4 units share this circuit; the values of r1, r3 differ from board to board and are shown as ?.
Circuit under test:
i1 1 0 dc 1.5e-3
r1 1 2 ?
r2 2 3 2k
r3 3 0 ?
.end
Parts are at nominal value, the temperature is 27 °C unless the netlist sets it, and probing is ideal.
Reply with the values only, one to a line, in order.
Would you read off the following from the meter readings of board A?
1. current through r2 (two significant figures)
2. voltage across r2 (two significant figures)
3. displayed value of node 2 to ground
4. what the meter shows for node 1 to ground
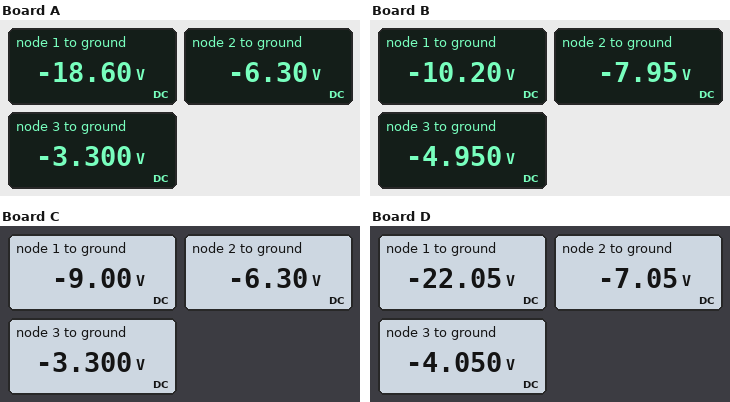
1.5 mA
3.0 V
-6.30 V
-18.60 V
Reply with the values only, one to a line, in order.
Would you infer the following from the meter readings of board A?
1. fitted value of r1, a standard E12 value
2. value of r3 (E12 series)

8.2 kΩ
2.2 kΩ
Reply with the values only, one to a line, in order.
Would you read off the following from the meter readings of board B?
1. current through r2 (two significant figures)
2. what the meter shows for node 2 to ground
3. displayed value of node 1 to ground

1.5 mA
-7.95 V
-10.20 V
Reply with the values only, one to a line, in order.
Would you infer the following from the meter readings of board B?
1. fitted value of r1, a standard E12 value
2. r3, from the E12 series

1.5 kΩ
3.3 kΩ
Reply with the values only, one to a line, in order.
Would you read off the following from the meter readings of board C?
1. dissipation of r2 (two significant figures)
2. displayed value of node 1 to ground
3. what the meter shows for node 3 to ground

4.5 mW
-9.00 V
-3.300 V
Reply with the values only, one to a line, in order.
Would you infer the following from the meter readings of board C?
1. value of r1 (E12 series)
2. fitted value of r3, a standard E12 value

1.8 kΩ
2.2 kΩ
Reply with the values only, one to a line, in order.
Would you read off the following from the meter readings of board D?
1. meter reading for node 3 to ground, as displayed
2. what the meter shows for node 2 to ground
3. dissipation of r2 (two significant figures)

-4.050 V
-7.05 V
4.5 mW
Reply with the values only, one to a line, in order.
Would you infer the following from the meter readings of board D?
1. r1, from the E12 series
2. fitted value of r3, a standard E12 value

10 kΩ
2.7 kΩ
